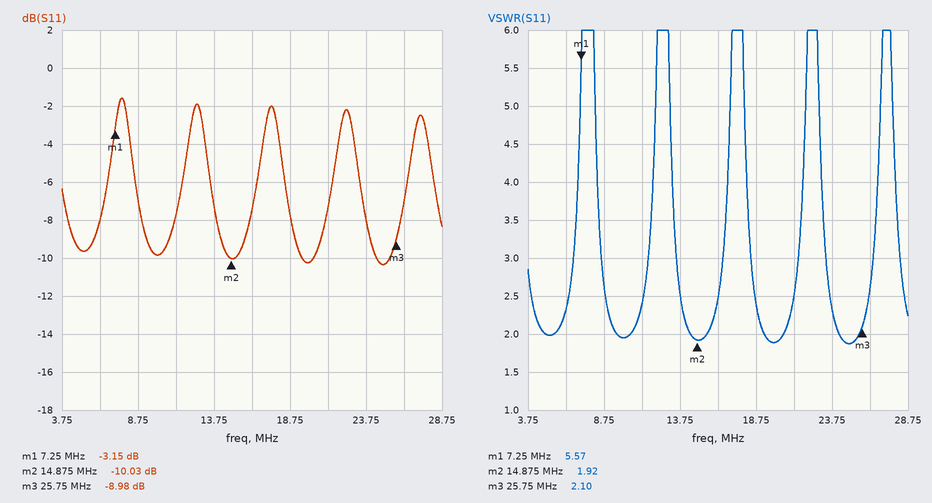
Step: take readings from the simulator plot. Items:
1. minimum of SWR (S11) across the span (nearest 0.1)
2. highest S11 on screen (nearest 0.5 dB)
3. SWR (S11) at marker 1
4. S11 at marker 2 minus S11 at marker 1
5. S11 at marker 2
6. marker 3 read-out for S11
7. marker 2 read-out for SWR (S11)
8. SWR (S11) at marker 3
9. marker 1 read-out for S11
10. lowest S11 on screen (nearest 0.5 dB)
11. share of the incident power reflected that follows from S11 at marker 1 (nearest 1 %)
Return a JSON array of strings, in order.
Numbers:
["1.9", "-1.5 dB", "5.57", "-6.88 dB", "-10.03 dB", "-8.98 dB", "1.92", "2.10", "-3.15 dB", "-10.5 dB", "48 %"]
